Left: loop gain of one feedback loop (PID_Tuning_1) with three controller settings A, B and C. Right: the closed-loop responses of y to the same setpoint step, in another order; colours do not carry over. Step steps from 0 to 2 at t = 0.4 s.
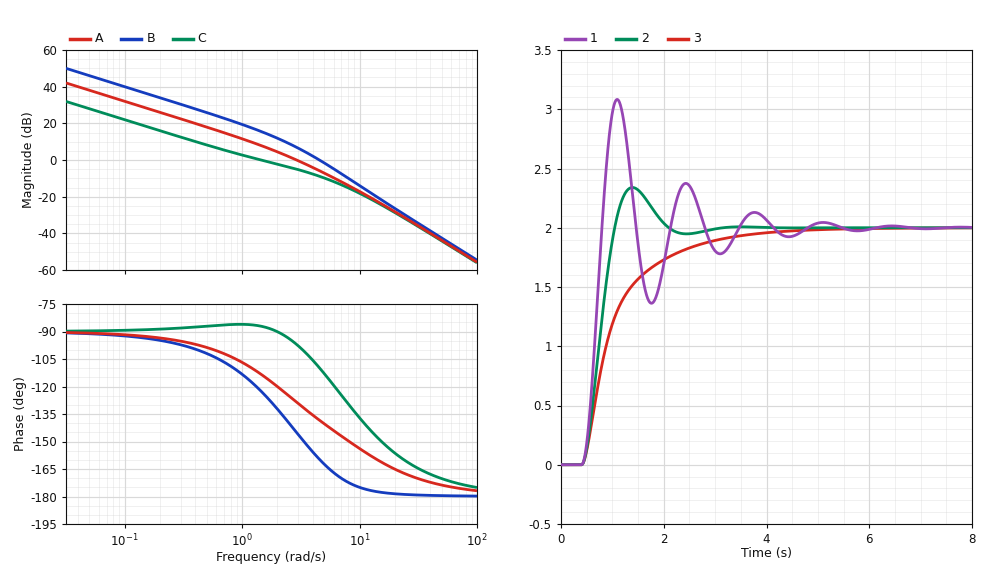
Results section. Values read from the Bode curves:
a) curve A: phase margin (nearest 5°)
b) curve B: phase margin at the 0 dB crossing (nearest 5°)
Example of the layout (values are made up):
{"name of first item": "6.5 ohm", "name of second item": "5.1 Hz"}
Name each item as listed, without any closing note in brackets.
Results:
{"curve A: phase margin": "50°", "curve B: phase margin at the 0 dB crossing": "20°"}
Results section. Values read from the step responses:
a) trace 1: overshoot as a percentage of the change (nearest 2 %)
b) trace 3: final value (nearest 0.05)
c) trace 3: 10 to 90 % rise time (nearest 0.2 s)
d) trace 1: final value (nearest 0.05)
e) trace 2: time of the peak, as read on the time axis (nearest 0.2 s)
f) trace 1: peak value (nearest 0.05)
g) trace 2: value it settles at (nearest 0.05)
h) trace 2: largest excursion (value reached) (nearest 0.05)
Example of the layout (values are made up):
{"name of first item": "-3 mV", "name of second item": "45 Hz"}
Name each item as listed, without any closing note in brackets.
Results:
{"trace 1: overshoot as a percentage of the change": "54 %", "trace 3: final value": "2.00", "trace 3: 10 to 90 % rise time": "1.8 s", "trace 1: final value": "2.00", "trace 2: time of the peak, as read on the time axis": "1.4 s", "trace 1: peak value": "3.10", "trace 2: value it settles at": "2.00", "trace 2: largest excursion (value reached)": "2.35"}
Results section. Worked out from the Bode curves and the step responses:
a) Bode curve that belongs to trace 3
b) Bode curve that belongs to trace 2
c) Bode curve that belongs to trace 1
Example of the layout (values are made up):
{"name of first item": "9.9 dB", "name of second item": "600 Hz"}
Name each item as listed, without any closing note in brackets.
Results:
{"Bode curve that belongs to trace 3": "C", "Bode curve that belongs to trace 2": "A", "Bode curve that belongs to trace 1": "B"}
